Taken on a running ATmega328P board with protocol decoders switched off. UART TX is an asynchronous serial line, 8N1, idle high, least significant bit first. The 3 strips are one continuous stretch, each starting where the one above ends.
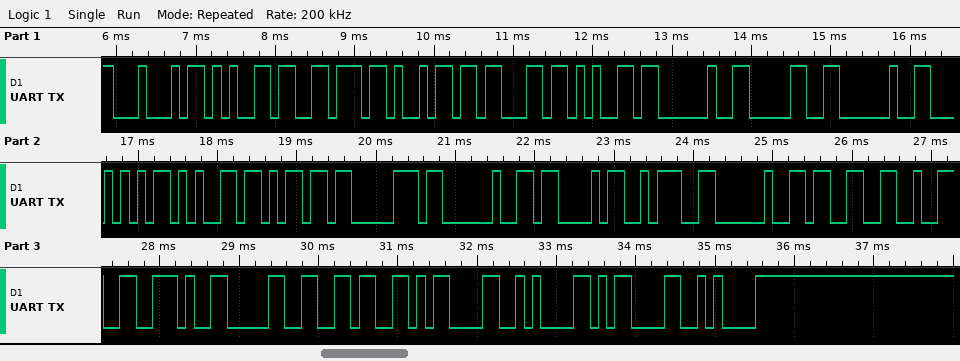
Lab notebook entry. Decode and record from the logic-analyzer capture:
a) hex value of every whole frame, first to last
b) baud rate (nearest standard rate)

44 65 76 69 63 65 20 30 20 54 65 6D 70 20 43 3A 20 33 32 2E 30 36 0D 0A 0D 0A
9600 baud
